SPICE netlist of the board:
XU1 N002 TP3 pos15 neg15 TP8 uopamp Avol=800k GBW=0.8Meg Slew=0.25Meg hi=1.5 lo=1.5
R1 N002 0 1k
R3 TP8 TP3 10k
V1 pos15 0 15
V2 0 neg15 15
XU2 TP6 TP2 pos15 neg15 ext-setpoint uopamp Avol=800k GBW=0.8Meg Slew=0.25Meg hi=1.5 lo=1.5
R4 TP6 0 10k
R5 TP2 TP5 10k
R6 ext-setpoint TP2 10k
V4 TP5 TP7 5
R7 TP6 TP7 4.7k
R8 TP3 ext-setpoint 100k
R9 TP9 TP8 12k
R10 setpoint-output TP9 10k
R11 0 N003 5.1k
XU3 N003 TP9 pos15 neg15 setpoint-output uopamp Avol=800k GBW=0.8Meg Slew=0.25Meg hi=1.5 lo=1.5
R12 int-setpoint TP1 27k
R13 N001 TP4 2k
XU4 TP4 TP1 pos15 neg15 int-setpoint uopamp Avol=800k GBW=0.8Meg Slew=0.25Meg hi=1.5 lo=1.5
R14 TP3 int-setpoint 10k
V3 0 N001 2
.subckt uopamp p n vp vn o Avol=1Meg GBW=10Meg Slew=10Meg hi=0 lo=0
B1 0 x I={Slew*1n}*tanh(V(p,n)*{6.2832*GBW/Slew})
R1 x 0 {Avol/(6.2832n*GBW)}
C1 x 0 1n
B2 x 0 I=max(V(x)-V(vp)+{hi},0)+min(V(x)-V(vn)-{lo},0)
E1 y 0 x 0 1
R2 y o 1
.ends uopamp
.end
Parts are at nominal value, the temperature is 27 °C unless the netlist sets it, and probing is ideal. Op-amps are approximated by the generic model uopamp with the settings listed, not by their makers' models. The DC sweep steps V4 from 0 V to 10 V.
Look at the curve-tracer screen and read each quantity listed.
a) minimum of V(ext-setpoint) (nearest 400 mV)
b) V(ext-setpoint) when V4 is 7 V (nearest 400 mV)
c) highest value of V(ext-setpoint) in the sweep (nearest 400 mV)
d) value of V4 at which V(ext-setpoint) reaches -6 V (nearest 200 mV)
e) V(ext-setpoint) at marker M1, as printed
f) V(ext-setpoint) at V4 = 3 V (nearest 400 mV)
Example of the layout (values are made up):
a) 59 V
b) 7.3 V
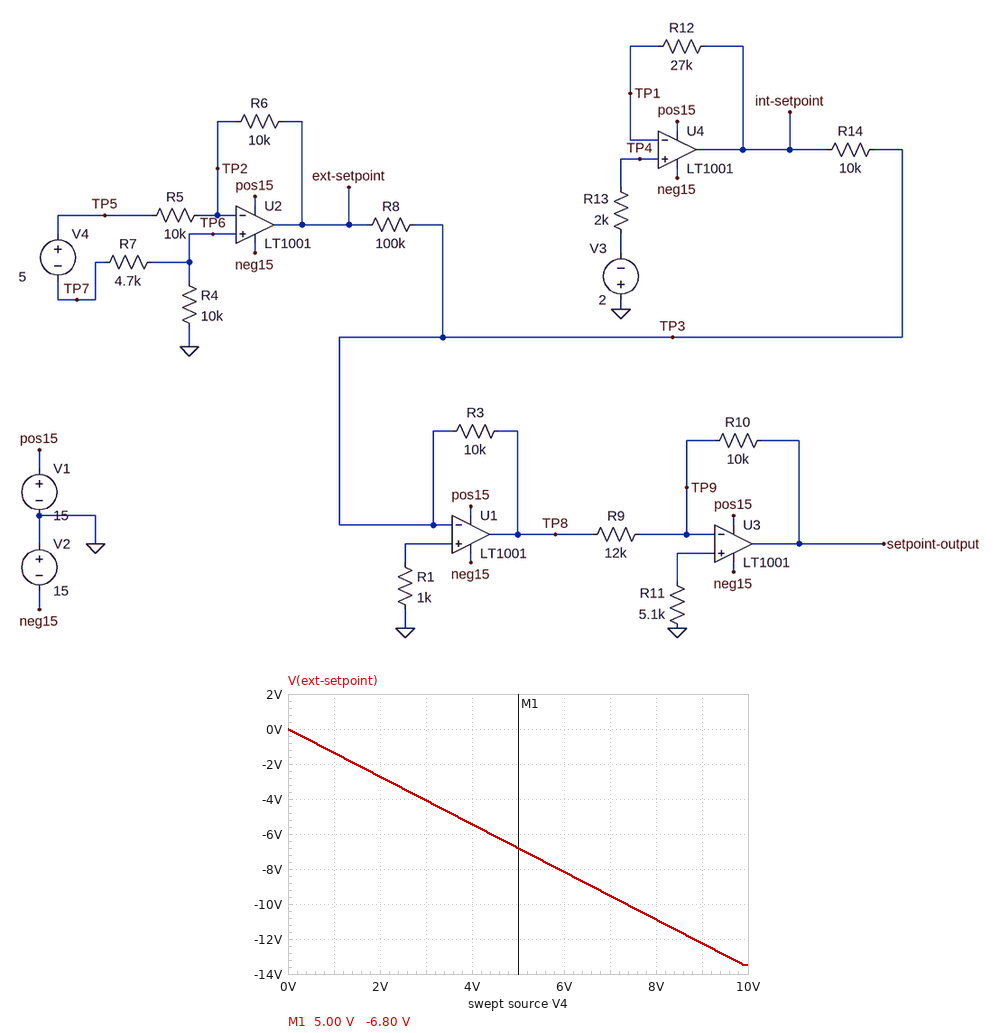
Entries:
a) -13.6 V
b) -9.6 V
c) 0 V
d) 4.4 V
e) -6.80 V
f) -4.0 V
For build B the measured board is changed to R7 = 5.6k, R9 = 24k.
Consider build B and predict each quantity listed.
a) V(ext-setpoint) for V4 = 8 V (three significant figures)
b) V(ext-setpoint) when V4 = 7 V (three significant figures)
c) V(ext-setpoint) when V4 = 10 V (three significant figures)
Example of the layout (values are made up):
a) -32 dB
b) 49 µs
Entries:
a) -10.3 V
b) -8.97 V
c) -12.8 V
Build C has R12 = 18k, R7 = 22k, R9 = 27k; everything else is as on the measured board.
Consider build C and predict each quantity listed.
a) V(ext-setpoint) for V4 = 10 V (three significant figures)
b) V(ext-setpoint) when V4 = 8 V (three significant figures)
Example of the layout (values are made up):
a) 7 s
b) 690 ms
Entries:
a) -6.25 V
b) -5.00 V
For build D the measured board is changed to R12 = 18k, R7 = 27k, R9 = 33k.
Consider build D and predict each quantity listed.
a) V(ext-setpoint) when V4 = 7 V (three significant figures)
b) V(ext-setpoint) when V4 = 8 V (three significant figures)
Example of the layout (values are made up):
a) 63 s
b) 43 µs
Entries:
a) -3.78 V
b) -4.32 V
